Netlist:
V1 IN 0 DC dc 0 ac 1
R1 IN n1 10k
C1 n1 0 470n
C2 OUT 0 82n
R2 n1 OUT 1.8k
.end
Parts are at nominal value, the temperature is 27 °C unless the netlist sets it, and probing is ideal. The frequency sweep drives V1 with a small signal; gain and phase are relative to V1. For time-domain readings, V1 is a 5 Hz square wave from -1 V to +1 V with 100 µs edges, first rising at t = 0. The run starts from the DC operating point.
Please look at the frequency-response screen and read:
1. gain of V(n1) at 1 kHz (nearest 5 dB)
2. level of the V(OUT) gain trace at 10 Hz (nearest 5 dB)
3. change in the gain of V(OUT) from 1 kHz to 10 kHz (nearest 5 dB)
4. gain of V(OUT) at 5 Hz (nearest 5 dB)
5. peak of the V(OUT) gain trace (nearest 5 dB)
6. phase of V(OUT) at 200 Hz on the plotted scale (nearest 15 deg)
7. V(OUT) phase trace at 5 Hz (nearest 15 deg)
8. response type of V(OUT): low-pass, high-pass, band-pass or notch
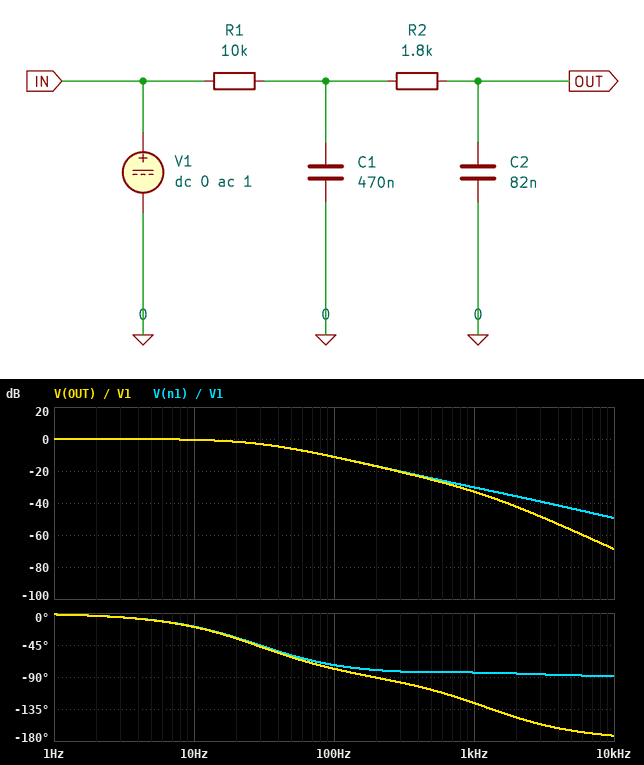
-30 dB
0 dB
-35 dB
0 dB
0 dB
-90 deg
-15 deg
low-pass
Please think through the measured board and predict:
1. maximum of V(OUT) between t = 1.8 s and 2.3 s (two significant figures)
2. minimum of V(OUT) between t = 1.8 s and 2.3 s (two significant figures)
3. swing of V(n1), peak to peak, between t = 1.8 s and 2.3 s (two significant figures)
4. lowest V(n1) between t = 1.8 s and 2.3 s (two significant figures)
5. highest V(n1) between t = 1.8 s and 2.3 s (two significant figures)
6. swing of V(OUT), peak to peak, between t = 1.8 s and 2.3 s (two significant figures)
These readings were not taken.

1.0 V
-1.0 V
2.0 V
-1.0 V
1.0 V
2.0 V
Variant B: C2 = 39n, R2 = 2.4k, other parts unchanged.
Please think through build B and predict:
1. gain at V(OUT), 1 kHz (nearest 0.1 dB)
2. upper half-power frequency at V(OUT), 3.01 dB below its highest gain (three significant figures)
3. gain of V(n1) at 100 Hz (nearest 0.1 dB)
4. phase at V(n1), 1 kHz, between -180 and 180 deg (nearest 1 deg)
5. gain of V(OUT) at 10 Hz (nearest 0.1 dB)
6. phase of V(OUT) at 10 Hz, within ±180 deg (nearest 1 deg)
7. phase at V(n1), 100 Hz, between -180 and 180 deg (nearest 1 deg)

-31.2 dB
31.2 Hz
-10.5 dB
-86 deg
-0.4 dB
-18 deg
-72 deg
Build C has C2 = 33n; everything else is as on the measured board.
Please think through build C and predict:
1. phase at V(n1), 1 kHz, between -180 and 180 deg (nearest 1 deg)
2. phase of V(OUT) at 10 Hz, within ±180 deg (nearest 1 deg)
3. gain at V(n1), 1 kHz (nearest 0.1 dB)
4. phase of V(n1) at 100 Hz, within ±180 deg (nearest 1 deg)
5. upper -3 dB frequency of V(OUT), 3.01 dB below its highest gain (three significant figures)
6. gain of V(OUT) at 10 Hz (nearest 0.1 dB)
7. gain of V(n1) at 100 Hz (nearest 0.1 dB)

-87 deg
-18 deg
-29.9 dB
-72 deg
31.6 Hz
-0.4 dB
-10.4 dB
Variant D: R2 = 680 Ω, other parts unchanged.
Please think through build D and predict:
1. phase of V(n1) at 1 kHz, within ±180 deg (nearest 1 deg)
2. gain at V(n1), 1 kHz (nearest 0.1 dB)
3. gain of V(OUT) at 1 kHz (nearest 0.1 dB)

-86 deg
-30.7 dB
-31.2 dB
